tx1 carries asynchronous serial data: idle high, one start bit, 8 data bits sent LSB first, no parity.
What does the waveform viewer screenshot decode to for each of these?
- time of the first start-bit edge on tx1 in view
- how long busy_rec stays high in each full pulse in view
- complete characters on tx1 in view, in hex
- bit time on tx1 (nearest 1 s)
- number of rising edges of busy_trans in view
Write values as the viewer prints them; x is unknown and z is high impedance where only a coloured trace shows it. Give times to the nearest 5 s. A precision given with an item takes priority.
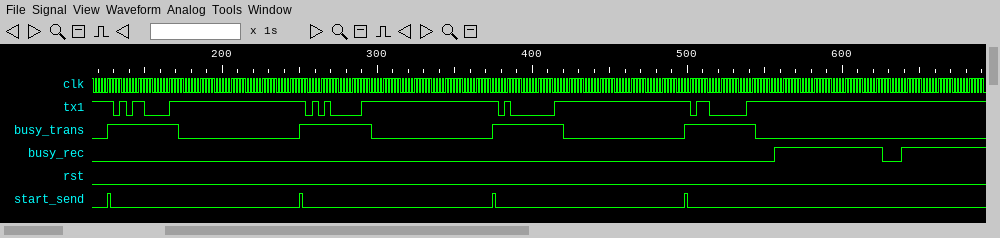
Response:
130 s
70 s
0D, 05, 01, 03
4 s
4
